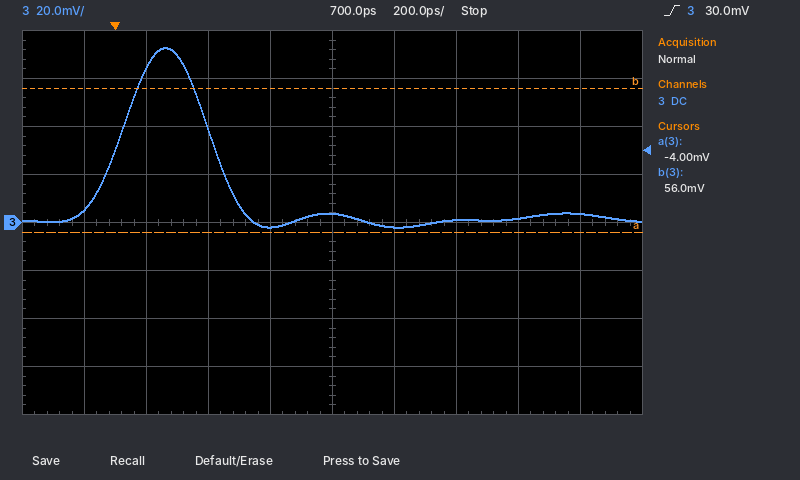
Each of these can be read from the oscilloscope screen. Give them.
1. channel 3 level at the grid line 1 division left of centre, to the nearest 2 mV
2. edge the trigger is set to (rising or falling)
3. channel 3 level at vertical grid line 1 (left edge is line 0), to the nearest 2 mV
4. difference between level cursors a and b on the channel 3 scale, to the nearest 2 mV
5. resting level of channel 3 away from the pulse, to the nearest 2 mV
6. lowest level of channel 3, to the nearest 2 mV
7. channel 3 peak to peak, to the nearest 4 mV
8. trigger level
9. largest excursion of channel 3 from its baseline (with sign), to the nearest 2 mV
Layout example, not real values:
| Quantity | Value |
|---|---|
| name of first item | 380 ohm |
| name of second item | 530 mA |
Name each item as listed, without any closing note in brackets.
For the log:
| Quantity | Value |
|---|---|
| channel 3 level at the grid line 1 division left of centre, to the nearest 2 mV | -2 mV |
| edge the trigger is set to | rising |
| channel 3 level at vertical grid line 1 (left edge is line 0), to the nearest 2 mV | 6 mV |
| difference between level cursors a and b on the channel 3 scale, to the nearest 2 mV | 60 mV |
| resting level of channel 3 away from the pulse, to the nearest 2 mV | 2 mV |
| lowest level of channel 3, to the nearest 2 mV | -2 mV |
| channel 3 peak to peak, to the nearest 4 mV | 76 mV |
| trigger level | 30.0 mV |
| largest excursion of channel 3 from its baseline (with sign), to the nearest 2 mV | +72 mV |
